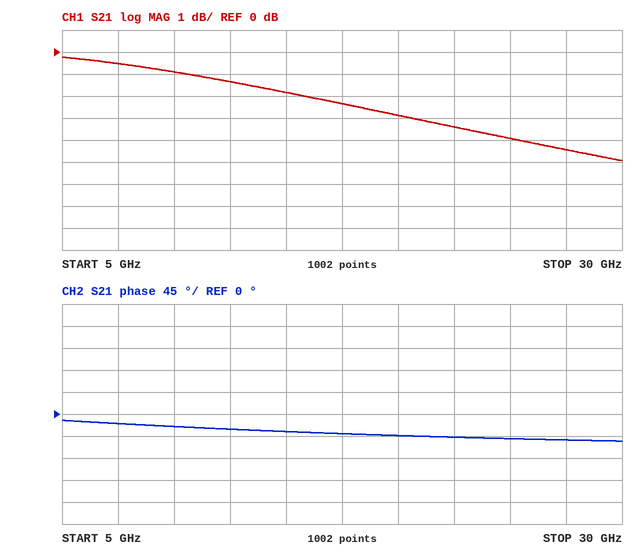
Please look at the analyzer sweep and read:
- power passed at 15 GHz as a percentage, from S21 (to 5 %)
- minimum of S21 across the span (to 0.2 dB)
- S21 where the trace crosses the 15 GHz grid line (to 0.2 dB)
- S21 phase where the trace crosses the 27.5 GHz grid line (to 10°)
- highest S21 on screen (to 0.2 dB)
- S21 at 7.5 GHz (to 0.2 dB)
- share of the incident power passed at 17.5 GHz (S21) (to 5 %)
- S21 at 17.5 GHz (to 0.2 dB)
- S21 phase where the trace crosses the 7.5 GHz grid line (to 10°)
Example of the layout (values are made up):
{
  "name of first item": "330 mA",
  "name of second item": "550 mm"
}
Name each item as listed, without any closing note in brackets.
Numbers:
{
  "power passed at 15 GHz as a percentage, from S21": "65 %",
  "minimum of S21 across the span": "-5.0 dB",
  "S21 where the trace crosses the 15 GHz grid line": "-1.8 dB",
  "S21 phase where the trace crosses the 27.5 GHz grid line": "-50°",
  "highest S21 on screen": "-0.2 dB",
  "S21 at 7.5 GHz": "-0.6 dB",
  "share of the incident power passed at 17.5 GHz (S21)": "60 %",
  "S21 at 17.5 GHz": "-2.4 dB",
  "S21 phase where the trace crosses the 7.5 GHz grid line": "-20°"
}
